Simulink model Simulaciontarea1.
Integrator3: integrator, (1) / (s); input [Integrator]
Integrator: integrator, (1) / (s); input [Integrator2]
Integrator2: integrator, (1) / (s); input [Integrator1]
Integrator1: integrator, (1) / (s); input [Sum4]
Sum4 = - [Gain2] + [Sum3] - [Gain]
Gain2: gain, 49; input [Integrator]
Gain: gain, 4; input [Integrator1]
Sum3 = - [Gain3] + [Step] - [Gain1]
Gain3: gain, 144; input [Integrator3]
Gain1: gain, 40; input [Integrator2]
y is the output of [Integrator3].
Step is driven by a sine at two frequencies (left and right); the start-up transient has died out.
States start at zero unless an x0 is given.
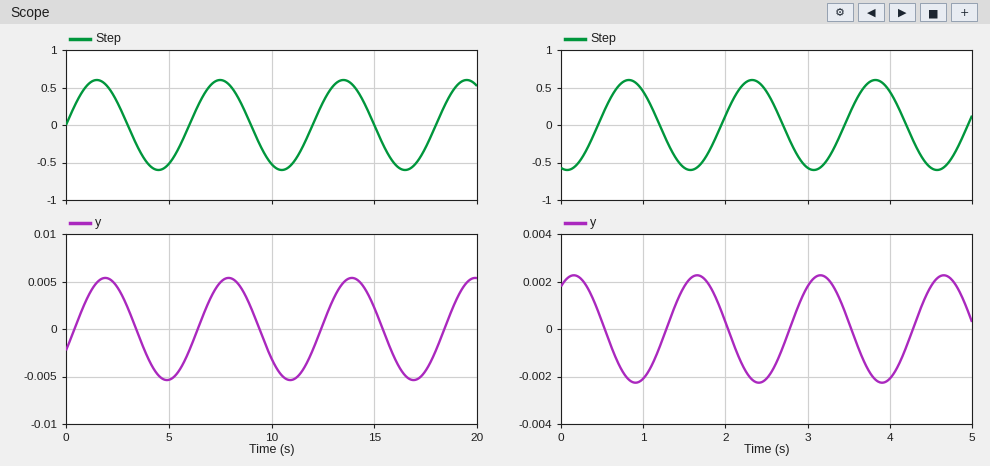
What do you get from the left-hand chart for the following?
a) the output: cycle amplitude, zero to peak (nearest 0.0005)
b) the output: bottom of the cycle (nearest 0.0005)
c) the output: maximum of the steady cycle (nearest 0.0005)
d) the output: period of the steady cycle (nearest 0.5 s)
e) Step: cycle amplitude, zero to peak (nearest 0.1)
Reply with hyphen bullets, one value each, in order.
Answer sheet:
- 0.0055
- -0.0055
- 0.0055
- 6.0 s
- 0.6
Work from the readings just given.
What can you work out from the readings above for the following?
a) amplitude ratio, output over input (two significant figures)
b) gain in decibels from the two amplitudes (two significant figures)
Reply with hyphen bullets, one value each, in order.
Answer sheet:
- 0.0092
- -41 dB
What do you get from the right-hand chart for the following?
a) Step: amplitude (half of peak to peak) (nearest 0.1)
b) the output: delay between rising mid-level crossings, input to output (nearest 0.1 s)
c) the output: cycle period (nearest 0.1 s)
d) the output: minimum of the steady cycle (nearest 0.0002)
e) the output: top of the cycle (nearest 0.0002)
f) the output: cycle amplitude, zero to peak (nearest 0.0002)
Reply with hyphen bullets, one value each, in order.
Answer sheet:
- 0.6
- 0.8 s
- 1.5 s
- -0.0022
- 0.0022
- 0.0022
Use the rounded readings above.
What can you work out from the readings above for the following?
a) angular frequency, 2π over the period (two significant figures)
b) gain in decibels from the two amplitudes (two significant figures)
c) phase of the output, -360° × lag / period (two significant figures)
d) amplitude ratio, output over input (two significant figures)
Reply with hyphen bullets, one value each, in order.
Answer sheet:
- 4.2 rad/s
- -49 dB
- -190°
- 0.0037
